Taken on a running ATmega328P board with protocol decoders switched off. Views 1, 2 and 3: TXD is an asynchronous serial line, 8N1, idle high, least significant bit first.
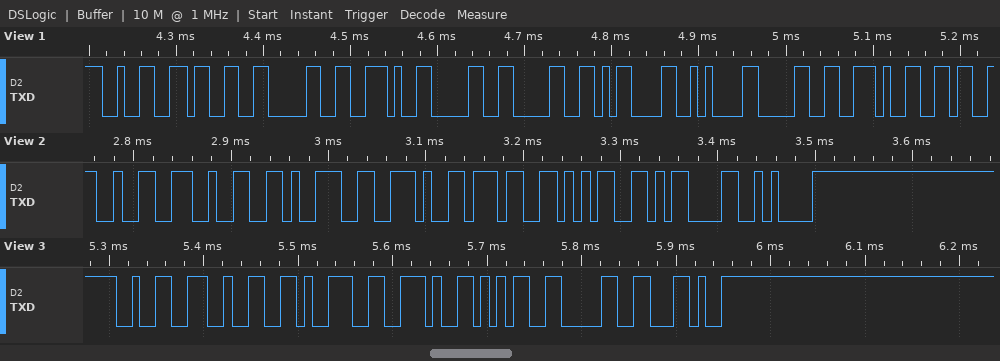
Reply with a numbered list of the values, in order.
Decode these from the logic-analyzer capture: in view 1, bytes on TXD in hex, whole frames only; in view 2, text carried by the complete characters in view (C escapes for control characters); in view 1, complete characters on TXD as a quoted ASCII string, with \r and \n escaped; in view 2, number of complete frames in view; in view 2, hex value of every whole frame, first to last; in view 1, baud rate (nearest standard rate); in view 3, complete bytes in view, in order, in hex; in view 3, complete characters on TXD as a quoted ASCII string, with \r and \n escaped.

1. 0x32 0x33 0x30 0x2E 0x30 0x30 0x0D 0x0A 0x30 0x2E 0x36
2. "229.75\r\n"
3. "230.00\r\n0.6"
4. 8
5. 0x32 0x32 0x39 0x2E 0x37 0x35 0x0D 0x0A
6. 115200 baud
7. 0x32 0x32 0x39 0x2E 0x35 0x30 0x2C
8. "229.50,"
